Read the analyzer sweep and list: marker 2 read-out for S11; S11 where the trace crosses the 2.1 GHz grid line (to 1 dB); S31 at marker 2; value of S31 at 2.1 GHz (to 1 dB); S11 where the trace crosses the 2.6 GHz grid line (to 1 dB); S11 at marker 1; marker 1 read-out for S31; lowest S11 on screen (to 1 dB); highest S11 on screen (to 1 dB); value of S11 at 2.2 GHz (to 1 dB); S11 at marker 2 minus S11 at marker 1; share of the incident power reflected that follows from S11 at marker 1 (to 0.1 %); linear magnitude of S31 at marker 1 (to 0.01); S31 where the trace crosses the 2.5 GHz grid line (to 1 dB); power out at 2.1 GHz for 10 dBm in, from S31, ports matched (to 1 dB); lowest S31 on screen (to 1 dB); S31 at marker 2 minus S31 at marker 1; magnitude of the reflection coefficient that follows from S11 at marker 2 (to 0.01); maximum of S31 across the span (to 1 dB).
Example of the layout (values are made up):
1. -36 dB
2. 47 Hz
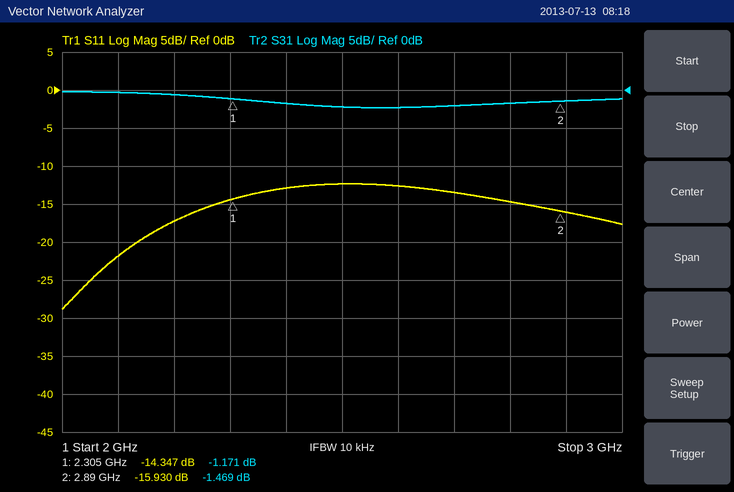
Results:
1. -15.930 dB
2. -22 dB
3. -1.469 dB
4. 0 dB
5. -13 dB
6. -14.347 dB
7. -1.171 dB
8. -29 dB
9. -12 dB
10. -17 dB
11. -1.583 dB
12. 3.7 %
13. 0.87
14. -2 dB
15. 10 dBm
16. -2 dB
17. -0.298 dB
18. 0.16
19. 0 dB
